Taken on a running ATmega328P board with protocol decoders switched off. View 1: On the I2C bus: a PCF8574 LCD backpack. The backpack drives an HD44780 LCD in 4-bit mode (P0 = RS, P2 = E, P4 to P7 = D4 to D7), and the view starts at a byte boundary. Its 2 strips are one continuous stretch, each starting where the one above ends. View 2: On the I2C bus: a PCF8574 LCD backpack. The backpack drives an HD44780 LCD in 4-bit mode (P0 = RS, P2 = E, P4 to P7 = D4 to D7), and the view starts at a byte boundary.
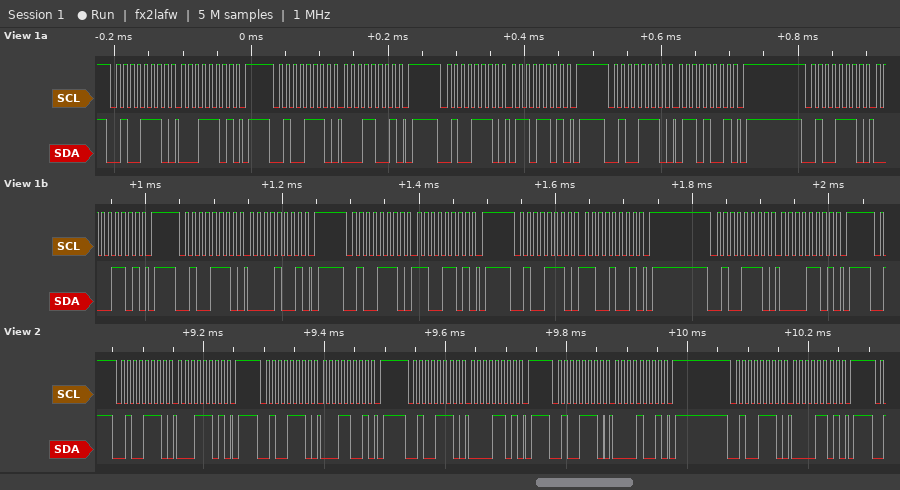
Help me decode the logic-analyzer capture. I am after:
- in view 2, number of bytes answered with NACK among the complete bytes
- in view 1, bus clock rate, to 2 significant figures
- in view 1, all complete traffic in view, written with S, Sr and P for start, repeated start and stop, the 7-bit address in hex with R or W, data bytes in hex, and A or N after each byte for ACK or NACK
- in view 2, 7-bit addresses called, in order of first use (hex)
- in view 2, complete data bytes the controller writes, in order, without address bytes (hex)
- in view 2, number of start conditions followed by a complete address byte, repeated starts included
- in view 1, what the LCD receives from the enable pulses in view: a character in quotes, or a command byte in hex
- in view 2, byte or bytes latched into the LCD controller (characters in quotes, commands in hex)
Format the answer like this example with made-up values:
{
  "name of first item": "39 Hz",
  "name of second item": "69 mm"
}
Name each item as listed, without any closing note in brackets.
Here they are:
{
  "in view 2, number of bytes answered with NACK among the complete bytes": "0",
  "in view 1, bus clock rate, to 2 significant figures": "100 kHz",
  "in view 1, all complete traffic in view, written with S, Sr and P for start, repeated start and stop, the 7-bit address in hex with R or W, data bytes in hex, and A or N after each byte for ACK or NACK": "S 27W A 1D A P S 27W A 19 A P S 27W A 6D A P S 27W A 69 A P S 27W A 0D A P S 27W A 09 A P S 27W A CD A P S 27W A C9 A P S 27W A 0D A P",
  "in view 2, 7-bit addresses called, in order of first use": "0x27",
  "in view 2, complete data bytes the controller writes, in order, without address bytes": "1D 19 0D 09 0D",
  "in view 2, number of start conditions followed by a complete address byte, repeated starts included": "5",
  "in view 1, what the LCD receives from the enable pulses in view: a character in quotes, or a command byte in hex": "data 0x16 data 0x0C",
  "in view 2, byte or bytes latched into the LCD controller": "data 0x10"
}
